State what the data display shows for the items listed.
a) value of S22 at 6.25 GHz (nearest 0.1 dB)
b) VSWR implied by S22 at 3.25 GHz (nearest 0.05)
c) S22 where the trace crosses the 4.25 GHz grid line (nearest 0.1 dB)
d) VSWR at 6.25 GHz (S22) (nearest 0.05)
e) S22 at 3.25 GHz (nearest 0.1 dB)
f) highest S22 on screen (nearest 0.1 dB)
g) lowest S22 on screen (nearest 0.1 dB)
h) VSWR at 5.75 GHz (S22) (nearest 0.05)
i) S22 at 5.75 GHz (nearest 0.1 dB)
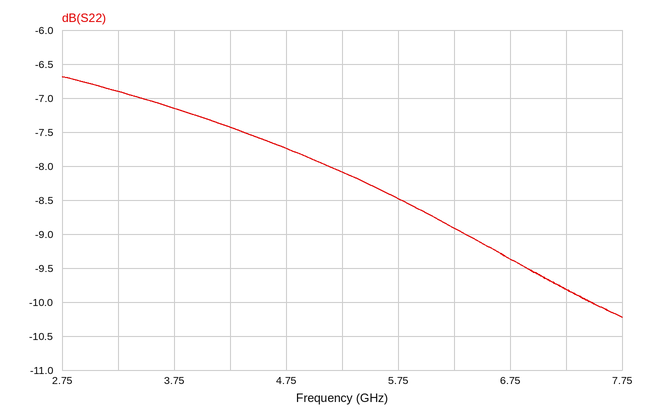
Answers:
-8.9 dB
2.65
-7.4 dB
2.10
-6.9 dB
-6.7 dB
-10.2 dB
2.20
-8.5 dB
